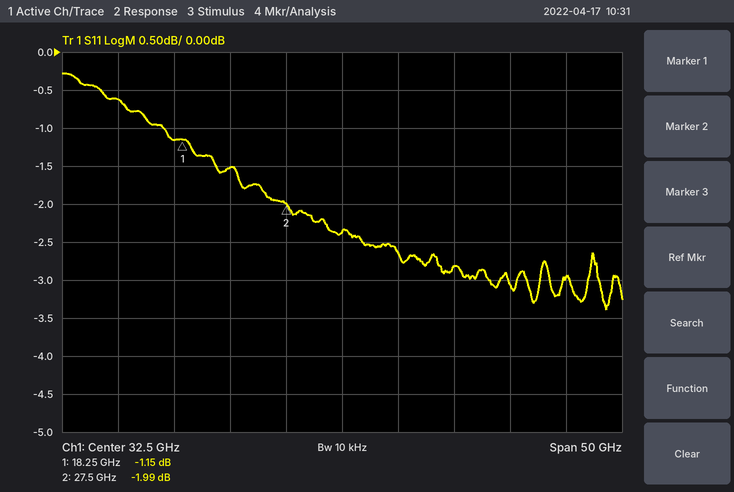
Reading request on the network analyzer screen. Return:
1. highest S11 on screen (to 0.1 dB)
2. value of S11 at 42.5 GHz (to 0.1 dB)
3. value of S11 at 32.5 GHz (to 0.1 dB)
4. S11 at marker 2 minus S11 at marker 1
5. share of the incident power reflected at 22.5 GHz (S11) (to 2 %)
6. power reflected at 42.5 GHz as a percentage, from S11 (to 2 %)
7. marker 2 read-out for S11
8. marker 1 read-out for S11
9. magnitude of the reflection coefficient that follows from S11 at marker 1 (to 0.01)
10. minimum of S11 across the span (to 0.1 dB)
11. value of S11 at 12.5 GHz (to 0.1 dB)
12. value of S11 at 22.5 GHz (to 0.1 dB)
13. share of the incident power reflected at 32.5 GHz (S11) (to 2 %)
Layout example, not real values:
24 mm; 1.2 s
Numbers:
-0.3 dB; -2.8 dB; -2.4 dB; -0.84 dB; 70 %; 52 %; -1.99 dB; -1.15 dB; 0.88; -3.4 dB; -0.6 dB; -1.5 dB; 58 %
